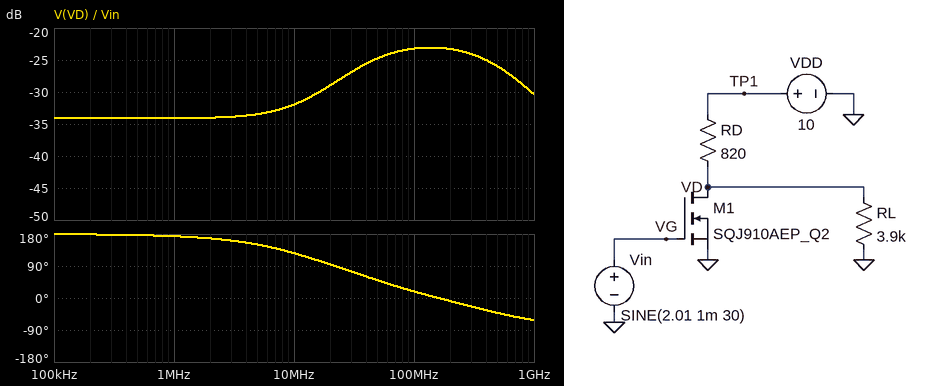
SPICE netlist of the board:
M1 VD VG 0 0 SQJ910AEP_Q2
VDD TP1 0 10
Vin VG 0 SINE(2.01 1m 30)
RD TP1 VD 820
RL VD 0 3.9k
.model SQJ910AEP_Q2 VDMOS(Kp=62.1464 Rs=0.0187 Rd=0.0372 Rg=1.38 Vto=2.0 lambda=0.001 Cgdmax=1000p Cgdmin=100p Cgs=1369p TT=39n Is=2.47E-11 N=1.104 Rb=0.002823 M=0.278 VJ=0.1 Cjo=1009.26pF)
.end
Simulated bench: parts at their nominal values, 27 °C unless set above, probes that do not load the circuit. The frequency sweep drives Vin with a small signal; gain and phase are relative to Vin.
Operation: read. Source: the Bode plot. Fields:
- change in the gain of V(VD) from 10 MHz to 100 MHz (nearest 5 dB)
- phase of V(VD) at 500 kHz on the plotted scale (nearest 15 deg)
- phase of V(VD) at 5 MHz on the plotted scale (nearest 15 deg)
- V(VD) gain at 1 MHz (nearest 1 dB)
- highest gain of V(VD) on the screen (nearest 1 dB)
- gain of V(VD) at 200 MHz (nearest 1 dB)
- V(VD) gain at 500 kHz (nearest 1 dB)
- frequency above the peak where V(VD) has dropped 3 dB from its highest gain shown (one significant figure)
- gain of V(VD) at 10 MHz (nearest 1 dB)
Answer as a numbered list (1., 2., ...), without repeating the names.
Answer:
1. 10 dB
2. 180 deg
3. 150 deg
4. -34 dB
5. -23 dB
6. -23 dB
7. -34 dB
8. 500 MHz
9. -32 dB
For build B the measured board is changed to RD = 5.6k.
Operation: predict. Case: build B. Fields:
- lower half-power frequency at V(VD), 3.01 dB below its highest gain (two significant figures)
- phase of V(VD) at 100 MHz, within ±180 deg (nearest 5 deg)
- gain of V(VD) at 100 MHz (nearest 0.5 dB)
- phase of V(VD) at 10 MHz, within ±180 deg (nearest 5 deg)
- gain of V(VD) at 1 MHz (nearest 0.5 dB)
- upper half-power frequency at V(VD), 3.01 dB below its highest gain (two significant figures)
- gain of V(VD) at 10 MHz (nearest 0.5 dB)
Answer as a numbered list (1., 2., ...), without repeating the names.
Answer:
1. 39 MHz
2. 15 deg
3. -23.5 dB
4. 85 deg
5. -50.0 dB
6. 520 MHz
7. -36.0 dB
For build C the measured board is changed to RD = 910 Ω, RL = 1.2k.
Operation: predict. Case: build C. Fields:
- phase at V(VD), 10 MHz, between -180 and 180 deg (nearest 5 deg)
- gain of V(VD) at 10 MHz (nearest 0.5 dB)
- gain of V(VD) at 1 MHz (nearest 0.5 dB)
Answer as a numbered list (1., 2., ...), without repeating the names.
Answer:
1. 125 deg
2. -32.5 dB
3. -35.0 dB
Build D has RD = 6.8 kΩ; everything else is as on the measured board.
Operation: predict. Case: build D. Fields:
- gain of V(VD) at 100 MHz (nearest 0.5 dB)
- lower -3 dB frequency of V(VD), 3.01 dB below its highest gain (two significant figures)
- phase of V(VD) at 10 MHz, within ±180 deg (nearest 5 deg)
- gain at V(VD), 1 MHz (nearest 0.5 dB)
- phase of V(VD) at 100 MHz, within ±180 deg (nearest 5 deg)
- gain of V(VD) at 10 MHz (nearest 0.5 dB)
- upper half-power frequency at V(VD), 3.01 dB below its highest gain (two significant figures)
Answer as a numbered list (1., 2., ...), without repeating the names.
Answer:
1. -23.5 dB
2. 39 MHz
3. 85 deg
4. -51.0 dB
5. 15 deg
6. -36.0 dB
7. 520 MHz
